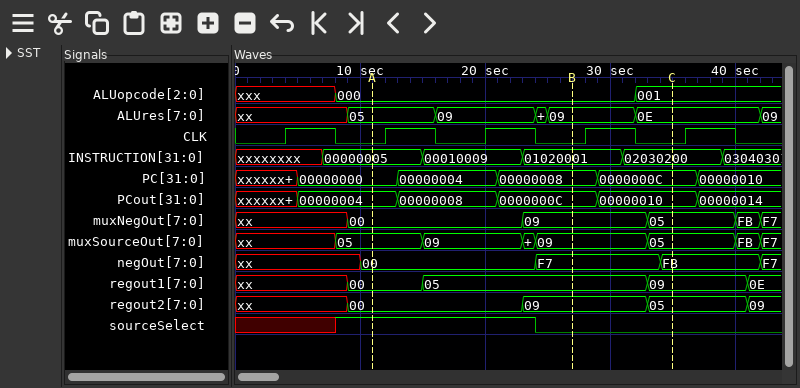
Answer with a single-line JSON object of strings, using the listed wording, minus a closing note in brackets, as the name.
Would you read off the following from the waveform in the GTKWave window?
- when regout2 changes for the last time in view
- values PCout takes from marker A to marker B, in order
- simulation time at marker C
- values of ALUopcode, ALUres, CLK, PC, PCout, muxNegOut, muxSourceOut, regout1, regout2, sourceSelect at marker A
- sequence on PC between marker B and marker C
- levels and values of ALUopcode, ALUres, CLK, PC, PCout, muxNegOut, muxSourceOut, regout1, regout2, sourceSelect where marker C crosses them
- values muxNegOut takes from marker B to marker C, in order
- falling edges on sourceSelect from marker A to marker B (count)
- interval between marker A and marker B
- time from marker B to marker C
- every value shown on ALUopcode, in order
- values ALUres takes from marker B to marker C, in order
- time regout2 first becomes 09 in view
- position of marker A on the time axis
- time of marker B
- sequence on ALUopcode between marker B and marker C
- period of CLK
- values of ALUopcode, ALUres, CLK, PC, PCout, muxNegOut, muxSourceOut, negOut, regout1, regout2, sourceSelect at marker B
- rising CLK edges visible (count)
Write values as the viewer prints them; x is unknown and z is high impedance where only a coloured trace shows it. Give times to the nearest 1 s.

{"when regout2 changes for the last time in view": "41 s", "values PCout takes from marker A to marker B, in order": "00000004, 00000008, 0000000C", "simulation time at marker C": "35 s", "values of ALUopcode, ALUres, CLK, PC, PCout, muxNegOut, muxSourceOut, regout1, regout2, sourceSelect at marker A": "ALUopcode=000, ALUres=05, CLK=0, PC=00000000, PCout=00000004, muxNegOut=00, muxSourceOut=05, regout1=00, regout2=00, sourceSelect=1", "sequence on PC between marker B and marker C": "00000008, 0000000C", "levels and values of ALUopcode, ALUres, CLK, PC, PCout, muxNegOut, muxSourceOut, regout1, regout2, sourceSelect where marker C crosses them": "ALUopcode=001, ALUres=0E, CLK=0, PC=0000000C, PCout=00000010, muxNegOut=05, muxSourceOut=05, regout1=09, regout2=05, sourceSelect=0", "values muxNegOut takes from marker B to marker C, in order": "09, 05", "falling edges on sourceSelect from marker A to marker B": "1", "interval between marker A and marker B": "16 s", "time from marker B to marker C": "8 s", "every value shown on ALUopcode, in order": "xxx, 000, 001", "values ALUres takes from marker B to marker C, in order": "09, 0E", "time regout2 first becomes 09 in view": "23 s", "position of marker A on the time axis": "11 s", "time of marker B": "27 s", "sequence on ALUopcode between marker B and marker C": "000, 001", "period of CLK": "8 s", "values of ALUopcode, ALUres, CLK, PC, PCout, muxNegOut, muxSourceOut, negOut, regout1, regout2, sourceSelect at marker B": "ALUopcode=000, ALUres=09, CLK=0, PC=00000008, PCout=0000000C, muxNegOut=09, muxSourceOut=09, negOut=F7, regout1=05, regout2=09, sourceSelect=0", "rising CLK edges visible": "5"}
